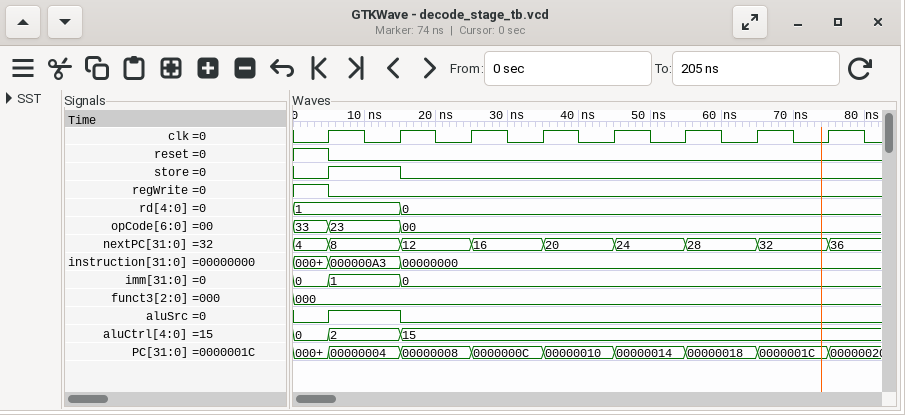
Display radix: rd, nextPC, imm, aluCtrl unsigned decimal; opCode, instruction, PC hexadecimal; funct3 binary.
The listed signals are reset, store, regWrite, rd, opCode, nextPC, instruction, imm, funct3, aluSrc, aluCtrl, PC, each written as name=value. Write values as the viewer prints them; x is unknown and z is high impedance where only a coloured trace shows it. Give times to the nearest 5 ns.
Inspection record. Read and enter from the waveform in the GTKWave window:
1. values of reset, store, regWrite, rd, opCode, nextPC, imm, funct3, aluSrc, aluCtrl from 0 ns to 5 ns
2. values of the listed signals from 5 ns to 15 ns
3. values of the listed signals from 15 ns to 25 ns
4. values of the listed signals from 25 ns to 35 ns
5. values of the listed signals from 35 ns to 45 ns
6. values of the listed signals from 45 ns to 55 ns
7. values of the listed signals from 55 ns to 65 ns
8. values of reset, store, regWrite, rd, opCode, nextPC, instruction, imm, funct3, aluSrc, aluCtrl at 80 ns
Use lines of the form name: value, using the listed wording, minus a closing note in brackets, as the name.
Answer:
values of reset, store, regWrite, rd, opCode, nextPC, imm, funct3, aluSrc, aluCtrl from 0 ns to 5 ns: reset=1, store=0, regWrite=1, rd=1, opCode=33, nextPC=4, imm=0, funct3=000, aluSrc=0, aluCtrl=0
values of the listed signals from 5 ns to 15 ns: reset=0, store=1, regWrite=0, rd=1, opCode=23, nextPC=8, instruction=000000A3, imm=1, funct3=000, aluSrc=1, aluCtrl=2, PC=00000004
values of the listed signals from 15 ns to 25 ns: reset=0, store=0, regWrite=0, rd=0, opCode=00, nextPC=12, instruction=00000000, imm=0, funct3=000, aluSrc=0, aluCtrl=15, PC=00000008
values of the listed signals from 25 ns to 35 ns: reset=0, store=0, regWrite=0, rd=0, opCode=00, nextPC=16, instruction=00000000, imm=0, funct3=000, aluSrc=0, aluCtrl=15, PC=0000000C
values of the listed signals from 35 ns to 45 ns: reset=0, store=0, regWrite=0, rd=0, opCode=00, nextPC=20, instruction=00000000, imm=0, funct3=000, aluSrc=0, aluCtrl=15, PC=00000010
values of the listed signals from 45 ns to 55 ns: reset=0, store=0, regWrite=0, rd=0, opCode=00, nextPC=24, instruction=00000000, imm=0, funct3=000, aluSrc=0, aluCtrl=15, PC=00000014
values of the listed signals from 55 ns to 65 ns: reset=0, store=0, regWrite=0, rd=0, opCode=00, nextPC=28, instruction=00000000, imm=0, funct3=000, aluSrc=0, aluCtrl=15, PC=00000018
values of reset, store, regWrite, rd, opCode, nextPC, instruction, imm, funct3, aluSrc, aluCtrl at 80 ns: reset=0, store=0, regWrite=0, rd=0, opCode=00, nextPC=36, instruction=00000000, imm=0, funct3=000, aluSrc=0, aluCtrl=15
